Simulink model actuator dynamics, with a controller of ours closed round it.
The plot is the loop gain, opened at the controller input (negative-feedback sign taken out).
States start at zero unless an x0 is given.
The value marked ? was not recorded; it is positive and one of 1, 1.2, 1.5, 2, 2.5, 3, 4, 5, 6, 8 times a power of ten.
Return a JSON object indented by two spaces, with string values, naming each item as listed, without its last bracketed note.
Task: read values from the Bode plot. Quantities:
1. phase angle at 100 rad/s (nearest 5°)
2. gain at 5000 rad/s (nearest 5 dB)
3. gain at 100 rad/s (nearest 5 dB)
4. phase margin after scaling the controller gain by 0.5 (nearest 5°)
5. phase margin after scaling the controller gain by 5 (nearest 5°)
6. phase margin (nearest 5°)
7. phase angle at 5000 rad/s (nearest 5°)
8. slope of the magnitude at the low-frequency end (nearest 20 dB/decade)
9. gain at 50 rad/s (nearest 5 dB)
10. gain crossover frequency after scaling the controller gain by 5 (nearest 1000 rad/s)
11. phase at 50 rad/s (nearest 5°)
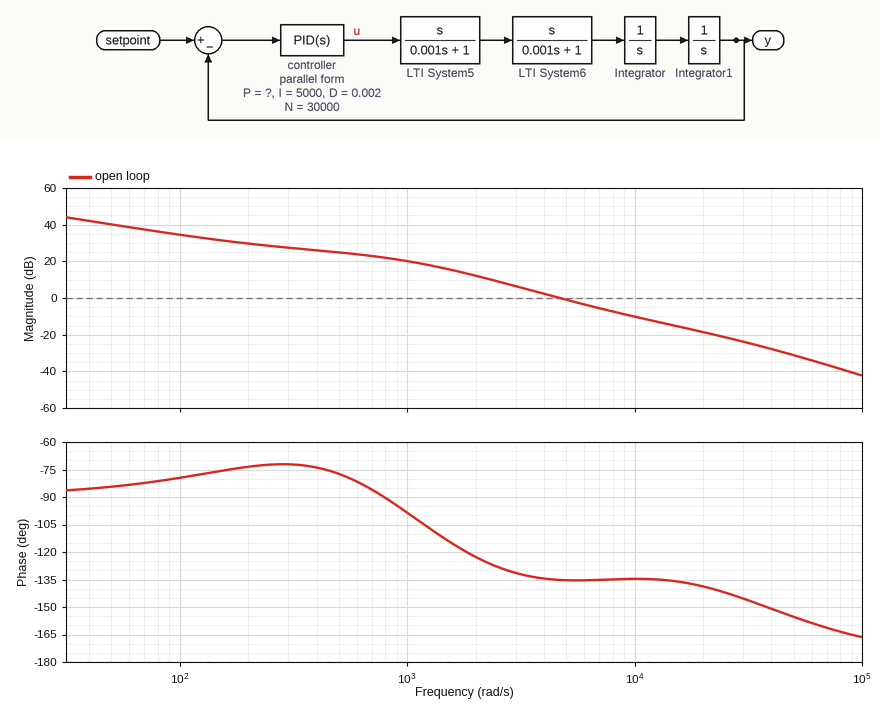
{
  "phase angle at 100 rad/s": "-80°",
  "gain at 5000 rad/s": "0 dB",
  "gain at 100 rad/s": "35 dB",
  "phase margin after scaling the controller gain by 0.5": "50°",
  "phase margin after scaling the controller gain by 5": "45°",
  "phase margin": "45°",
  "phase angle at 5000 rad/s": "-135°",
  "slope of the magnitude at the low-frequency end": "-20 dB/decade",
  "gain at 50 rad/s": "40 dB",
  "gain crossover frequency after scaling the controller gain by 5": "14000 rad/s",
  "phase at 50 rad/s": "-85°"
}
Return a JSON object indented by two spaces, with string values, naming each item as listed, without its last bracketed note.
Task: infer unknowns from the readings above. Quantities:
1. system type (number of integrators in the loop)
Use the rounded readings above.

{
  "system type": "1"
}
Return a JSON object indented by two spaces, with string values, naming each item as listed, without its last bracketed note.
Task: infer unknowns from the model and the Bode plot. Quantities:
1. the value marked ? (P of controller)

{
  "the value marked ?": "20"
}
